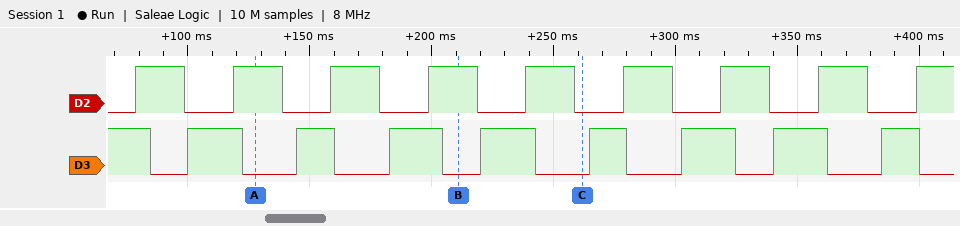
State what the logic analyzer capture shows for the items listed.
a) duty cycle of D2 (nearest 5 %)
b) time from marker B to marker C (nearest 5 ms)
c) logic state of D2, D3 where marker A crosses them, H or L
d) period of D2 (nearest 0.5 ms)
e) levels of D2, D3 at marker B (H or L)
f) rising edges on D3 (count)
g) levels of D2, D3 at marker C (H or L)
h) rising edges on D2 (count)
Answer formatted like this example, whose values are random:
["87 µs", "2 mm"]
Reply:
["50 %", "50 ms", "D2=H, D3=L", "40 ms", "D2=H, D3=L", "8", "D2=L, D3=L", "9"]
